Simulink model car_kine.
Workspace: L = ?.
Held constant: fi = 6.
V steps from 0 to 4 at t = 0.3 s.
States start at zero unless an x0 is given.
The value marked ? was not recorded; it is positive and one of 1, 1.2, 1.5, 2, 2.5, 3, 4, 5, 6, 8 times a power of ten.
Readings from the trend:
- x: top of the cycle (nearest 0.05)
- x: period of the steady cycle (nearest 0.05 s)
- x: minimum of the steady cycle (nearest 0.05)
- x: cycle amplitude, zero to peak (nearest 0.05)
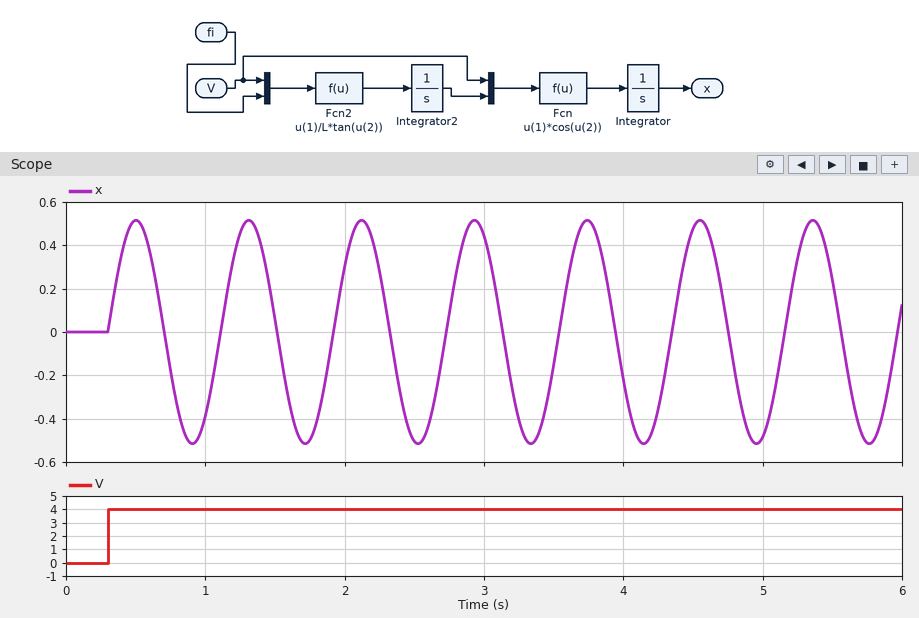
0.50
0.80 s
-0.50
0.50
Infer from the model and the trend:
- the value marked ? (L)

0.15
